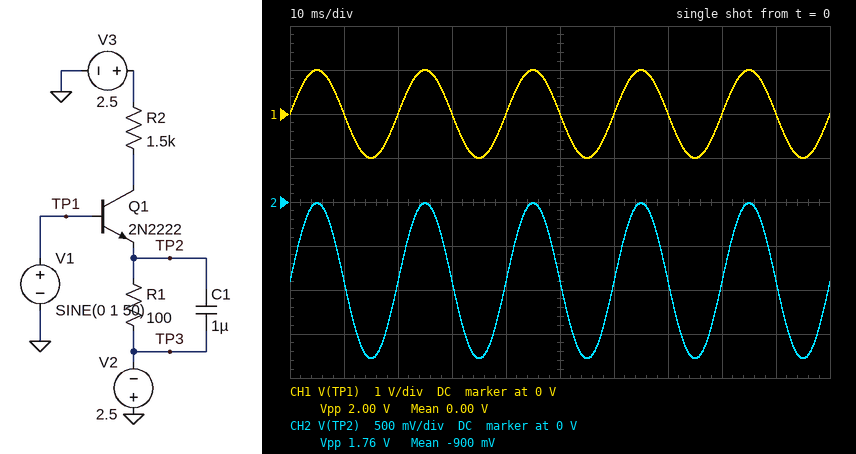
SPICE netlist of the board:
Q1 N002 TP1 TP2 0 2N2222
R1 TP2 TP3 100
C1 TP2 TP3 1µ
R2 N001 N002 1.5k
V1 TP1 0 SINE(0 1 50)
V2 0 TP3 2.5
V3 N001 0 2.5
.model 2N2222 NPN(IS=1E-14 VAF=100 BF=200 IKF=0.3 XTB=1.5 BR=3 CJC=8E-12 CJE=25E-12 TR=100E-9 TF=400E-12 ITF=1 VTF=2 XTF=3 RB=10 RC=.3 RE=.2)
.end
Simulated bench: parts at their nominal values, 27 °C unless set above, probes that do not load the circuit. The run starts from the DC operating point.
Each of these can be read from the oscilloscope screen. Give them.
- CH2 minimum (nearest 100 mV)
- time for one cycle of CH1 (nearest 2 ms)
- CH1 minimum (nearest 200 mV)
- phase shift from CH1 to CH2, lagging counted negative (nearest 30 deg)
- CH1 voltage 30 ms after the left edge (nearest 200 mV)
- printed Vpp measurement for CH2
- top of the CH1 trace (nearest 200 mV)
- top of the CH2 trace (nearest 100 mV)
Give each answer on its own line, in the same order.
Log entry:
-1.8 V
20 ms
-1.0 V
0 deg
0 V
1.76 V
1.0 V
0 V
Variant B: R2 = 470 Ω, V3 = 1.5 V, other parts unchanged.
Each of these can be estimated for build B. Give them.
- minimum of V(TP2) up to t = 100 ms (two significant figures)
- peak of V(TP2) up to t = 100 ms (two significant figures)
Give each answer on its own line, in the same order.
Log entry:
-1.7 V
3.2 mV
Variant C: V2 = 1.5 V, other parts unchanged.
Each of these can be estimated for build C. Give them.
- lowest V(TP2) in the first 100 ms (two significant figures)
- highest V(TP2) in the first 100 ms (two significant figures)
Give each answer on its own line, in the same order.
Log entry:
-1.5 V
92 mV
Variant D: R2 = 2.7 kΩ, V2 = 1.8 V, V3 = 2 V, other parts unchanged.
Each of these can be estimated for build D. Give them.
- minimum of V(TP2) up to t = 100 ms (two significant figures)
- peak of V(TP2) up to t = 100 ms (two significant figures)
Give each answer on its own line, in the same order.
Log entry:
-1.7 V
52 mV
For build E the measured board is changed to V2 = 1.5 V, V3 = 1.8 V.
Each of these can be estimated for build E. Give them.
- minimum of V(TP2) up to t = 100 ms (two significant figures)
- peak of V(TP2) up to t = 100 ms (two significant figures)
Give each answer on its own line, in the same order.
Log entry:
-1.5 V
88 mV
